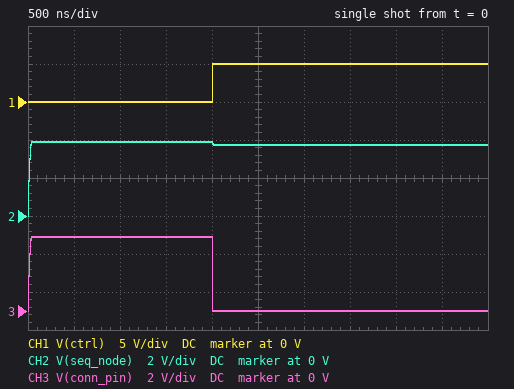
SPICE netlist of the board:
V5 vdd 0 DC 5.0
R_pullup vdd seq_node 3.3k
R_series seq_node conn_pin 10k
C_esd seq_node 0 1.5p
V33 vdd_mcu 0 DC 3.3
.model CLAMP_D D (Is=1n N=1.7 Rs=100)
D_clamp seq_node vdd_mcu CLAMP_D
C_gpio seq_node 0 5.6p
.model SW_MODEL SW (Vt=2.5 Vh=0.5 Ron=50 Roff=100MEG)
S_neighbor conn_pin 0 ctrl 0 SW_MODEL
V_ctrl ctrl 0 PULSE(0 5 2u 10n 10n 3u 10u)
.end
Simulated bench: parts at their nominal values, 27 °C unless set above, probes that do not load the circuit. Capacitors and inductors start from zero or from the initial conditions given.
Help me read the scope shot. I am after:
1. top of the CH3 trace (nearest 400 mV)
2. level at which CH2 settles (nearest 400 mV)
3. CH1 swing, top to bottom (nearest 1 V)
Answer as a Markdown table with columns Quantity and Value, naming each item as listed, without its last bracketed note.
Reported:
| Quantity | Value |
|---|---|
| top of the CH3 trace | 4.0 V |
| level at which CH2 settles | 3.6 V |
| CH1 swing, top to bottom | 5 V |
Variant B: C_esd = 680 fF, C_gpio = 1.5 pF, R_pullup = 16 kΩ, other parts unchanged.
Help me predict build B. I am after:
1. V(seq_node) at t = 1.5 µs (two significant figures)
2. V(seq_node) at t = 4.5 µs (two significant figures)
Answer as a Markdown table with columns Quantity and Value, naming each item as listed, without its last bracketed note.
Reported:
| Quantity | Value |
|---|---|
| V(seq_node) at t = 1.5 µs | 3.8 V |
| V(seq_node) at t = 4.5 µs | 1.9 V |
